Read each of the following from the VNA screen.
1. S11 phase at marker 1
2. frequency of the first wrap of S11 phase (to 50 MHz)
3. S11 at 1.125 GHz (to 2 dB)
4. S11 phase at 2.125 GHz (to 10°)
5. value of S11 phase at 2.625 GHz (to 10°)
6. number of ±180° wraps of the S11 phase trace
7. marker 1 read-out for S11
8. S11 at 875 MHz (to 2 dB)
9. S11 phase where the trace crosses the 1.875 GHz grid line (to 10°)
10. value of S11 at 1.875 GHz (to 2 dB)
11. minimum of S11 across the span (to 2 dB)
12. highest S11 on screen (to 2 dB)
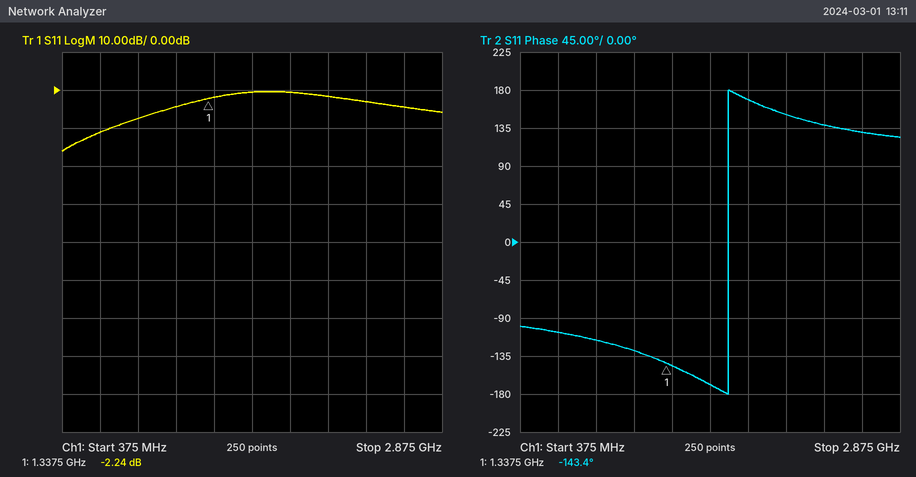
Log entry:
-143.4°
1.75 GHz
-4 dB
150°
130°
1
-2.24 dB
-8 dB
170°
0 dB
-16 dB
0 dB
